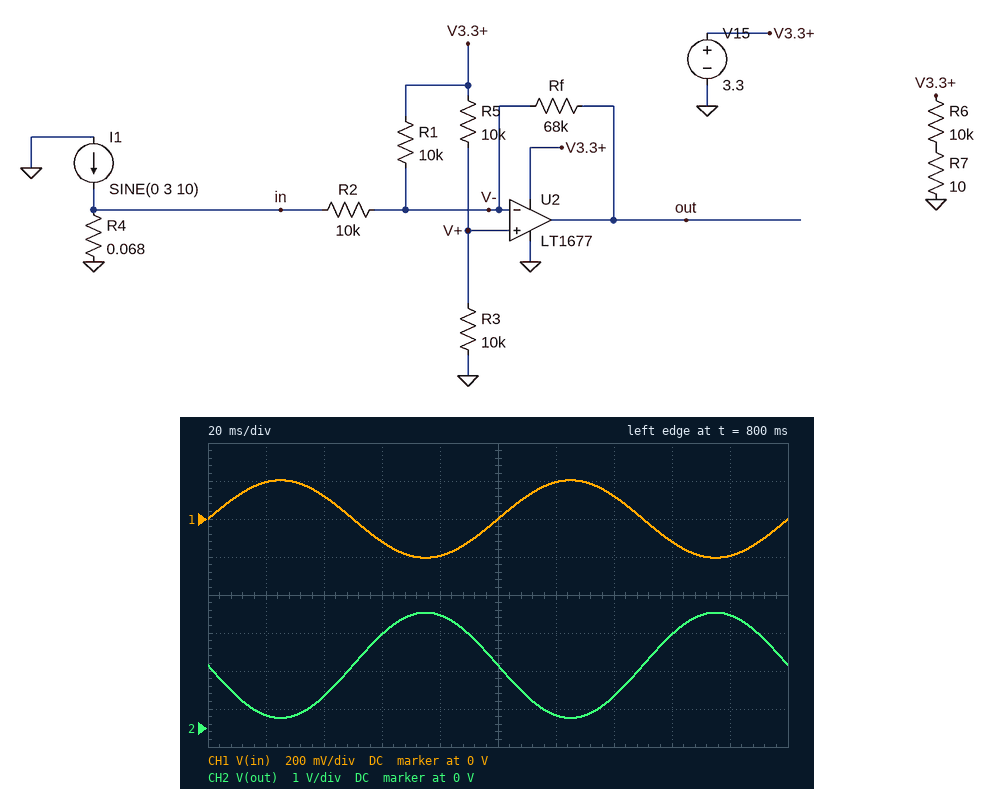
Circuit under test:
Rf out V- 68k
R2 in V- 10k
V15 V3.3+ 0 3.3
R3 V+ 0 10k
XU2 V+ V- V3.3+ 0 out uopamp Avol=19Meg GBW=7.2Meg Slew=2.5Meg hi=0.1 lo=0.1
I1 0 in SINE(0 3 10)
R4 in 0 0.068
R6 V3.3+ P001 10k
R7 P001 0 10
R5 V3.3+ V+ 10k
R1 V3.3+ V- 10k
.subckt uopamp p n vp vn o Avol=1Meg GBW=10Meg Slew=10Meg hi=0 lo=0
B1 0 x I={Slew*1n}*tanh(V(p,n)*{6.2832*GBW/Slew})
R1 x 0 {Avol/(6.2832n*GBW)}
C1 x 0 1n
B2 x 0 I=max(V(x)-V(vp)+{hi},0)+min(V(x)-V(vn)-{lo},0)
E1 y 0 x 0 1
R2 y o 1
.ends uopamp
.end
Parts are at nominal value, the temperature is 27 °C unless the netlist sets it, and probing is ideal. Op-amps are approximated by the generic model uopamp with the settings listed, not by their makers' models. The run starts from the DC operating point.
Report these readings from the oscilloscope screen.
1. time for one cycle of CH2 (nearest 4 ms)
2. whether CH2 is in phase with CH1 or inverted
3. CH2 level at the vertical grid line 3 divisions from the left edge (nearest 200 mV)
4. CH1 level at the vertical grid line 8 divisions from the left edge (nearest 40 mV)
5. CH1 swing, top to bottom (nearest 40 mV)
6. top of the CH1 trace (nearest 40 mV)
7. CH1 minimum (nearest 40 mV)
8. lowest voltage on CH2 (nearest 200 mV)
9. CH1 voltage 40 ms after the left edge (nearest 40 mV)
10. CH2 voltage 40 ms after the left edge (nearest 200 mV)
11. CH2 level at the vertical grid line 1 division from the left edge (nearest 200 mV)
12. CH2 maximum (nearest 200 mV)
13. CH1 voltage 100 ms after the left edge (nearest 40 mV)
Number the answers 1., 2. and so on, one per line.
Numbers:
1. 100 ms
2. inverted
3. 2.4 V
4. -120 mV
5. 400 mV
6. 200 mV
7. -200 mV
8. 200 mV
9. 120 mV
10. 800 mV
11. 400 mV
12. 3.0 V
13. 0 V
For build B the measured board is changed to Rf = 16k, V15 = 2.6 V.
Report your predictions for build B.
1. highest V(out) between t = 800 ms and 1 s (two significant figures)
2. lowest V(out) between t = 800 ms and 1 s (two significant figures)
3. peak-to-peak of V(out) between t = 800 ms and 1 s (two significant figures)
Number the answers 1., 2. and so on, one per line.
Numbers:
1. 1.6 V
2. 970 mV
3. 650 mV
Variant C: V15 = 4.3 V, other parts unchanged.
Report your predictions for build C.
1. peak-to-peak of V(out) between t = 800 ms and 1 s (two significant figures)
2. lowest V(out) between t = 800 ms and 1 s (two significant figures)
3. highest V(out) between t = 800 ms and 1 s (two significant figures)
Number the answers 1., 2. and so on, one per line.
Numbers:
1. 2.8 V
2. 760 mV
3. 3.5 V
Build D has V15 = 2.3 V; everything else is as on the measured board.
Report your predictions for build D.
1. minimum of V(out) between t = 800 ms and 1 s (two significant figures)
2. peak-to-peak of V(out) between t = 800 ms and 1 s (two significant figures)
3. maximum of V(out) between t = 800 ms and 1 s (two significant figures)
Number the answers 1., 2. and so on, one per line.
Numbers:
1. 99 mV
2. 2.1 V
3. 2.2 V
